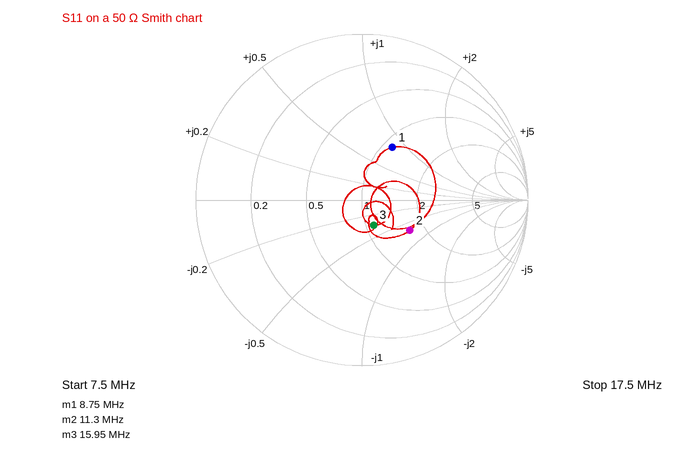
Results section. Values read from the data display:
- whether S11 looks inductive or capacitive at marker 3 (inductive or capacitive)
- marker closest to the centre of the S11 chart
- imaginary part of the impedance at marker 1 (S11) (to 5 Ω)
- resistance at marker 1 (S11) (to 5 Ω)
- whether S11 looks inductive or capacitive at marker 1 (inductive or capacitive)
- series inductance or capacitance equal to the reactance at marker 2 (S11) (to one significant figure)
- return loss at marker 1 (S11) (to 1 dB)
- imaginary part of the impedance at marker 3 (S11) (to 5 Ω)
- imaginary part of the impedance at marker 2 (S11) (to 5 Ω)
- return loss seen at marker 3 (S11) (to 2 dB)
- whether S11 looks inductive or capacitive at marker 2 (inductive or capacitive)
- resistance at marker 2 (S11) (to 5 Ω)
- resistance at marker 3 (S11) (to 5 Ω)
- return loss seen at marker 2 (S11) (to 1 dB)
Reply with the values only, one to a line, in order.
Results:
capacitive
marker 3
+40 Ω
55 Ω
inductive
400 pF
9 dB
-15 Ω
-35 Ω
16 dB
capacitive
80 Ω
55 Ω
9 dB
